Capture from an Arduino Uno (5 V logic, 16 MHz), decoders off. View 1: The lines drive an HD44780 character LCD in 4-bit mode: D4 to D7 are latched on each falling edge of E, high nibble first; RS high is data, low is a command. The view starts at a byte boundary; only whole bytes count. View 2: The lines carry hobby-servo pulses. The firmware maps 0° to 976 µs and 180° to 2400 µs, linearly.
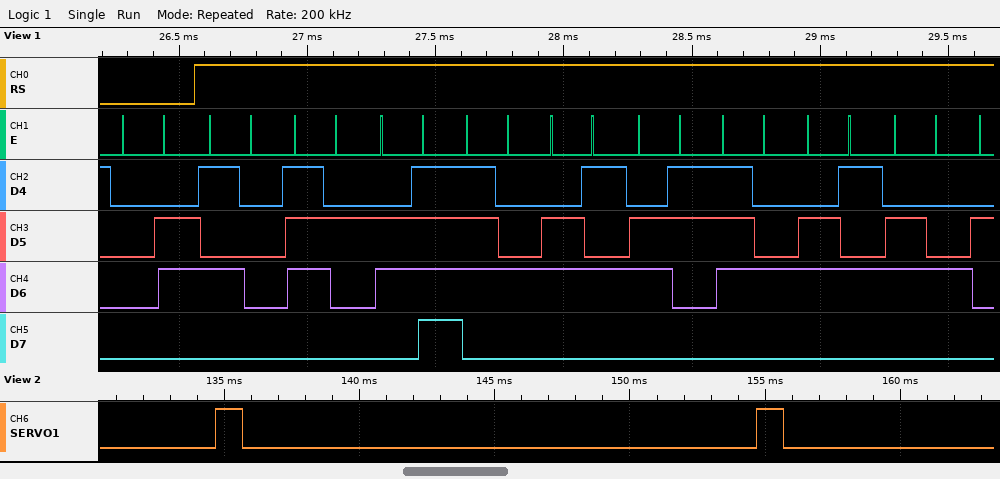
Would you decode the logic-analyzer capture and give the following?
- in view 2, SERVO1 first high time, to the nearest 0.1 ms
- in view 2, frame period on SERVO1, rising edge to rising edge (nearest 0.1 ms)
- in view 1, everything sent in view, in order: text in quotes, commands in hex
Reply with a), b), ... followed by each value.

a) 1.0 ms
b) 20.0 ms
c) 0x06 "Protected"
